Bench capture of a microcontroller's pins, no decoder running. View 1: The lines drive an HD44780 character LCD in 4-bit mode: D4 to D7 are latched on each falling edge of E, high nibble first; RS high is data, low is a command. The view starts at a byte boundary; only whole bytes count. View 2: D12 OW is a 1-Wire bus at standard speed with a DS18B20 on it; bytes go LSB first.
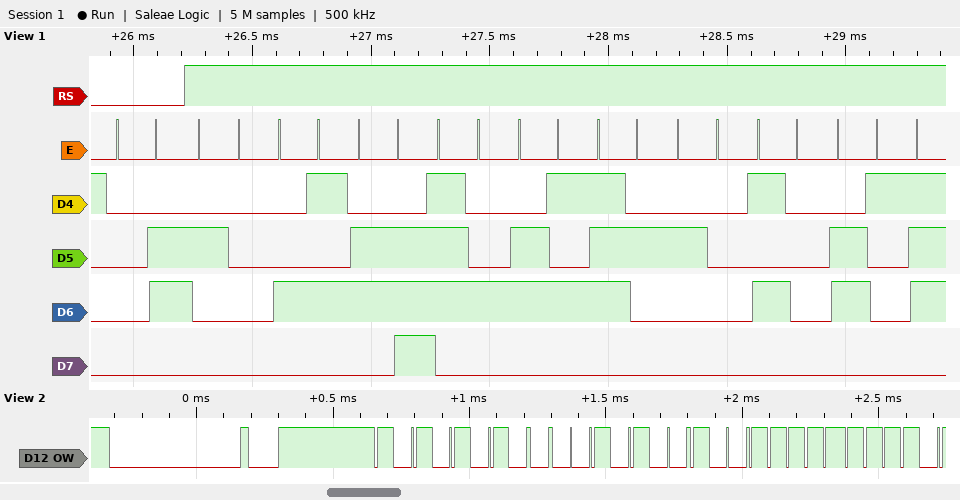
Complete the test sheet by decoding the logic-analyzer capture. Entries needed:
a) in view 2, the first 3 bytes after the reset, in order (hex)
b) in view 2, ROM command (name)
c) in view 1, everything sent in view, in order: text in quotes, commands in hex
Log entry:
55 28 F9
Match ROM
0x06 " Enter Pa"
